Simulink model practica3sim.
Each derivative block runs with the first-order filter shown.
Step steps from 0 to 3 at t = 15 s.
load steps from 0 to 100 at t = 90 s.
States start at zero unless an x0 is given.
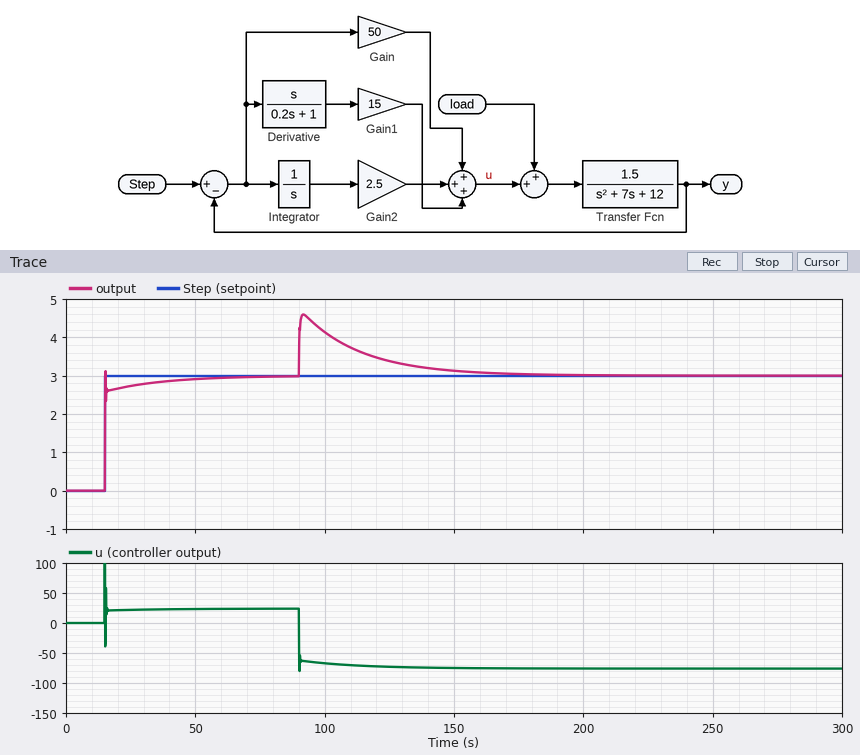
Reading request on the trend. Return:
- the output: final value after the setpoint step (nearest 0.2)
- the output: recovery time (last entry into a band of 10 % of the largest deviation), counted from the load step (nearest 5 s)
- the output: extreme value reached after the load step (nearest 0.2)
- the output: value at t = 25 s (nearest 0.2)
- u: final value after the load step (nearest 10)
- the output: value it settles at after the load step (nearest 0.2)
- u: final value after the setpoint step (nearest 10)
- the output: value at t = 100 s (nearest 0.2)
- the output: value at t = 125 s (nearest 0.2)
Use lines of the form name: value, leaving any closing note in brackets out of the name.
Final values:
the output: final value after the setpoint step: 3.0
the output: recovery time (last entry into a band of 10 % of the largest deviation), counted from the load step: 55 s
the output: extreme value reached after the load step: 4.6
the output: value at t = 25 s: 2.8
u: final value after the load step: -80
the output: value it settles at after the load step: 3.0
u: final value after the setpoint step: 20
the output: value at t = 100 s: 4.2
the output: value at t = 125 s: 3.4
